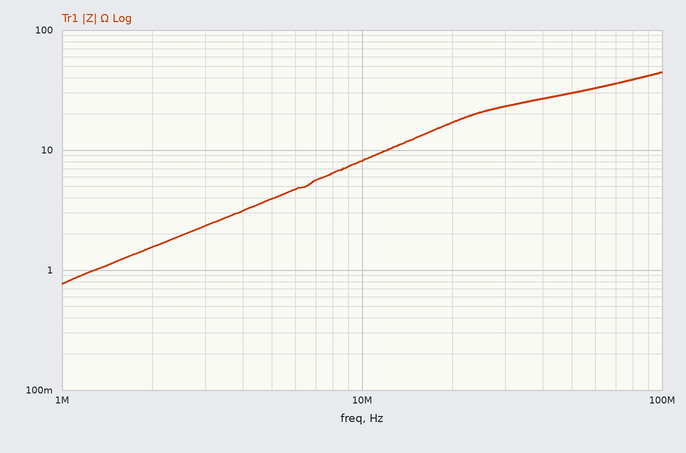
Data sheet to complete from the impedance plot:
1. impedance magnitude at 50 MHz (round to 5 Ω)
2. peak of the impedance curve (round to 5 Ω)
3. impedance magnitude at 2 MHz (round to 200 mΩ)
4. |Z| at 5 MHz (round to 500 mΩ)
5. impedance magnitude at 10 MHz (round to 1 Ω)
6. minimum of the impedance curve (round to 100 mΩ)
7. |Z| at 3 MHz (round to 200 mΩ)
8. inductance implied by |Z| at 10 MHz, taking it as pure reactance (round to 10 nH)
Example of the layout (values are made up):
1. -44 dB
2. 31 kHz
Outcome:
1. 30 Ω
2. 45 Ω
3. 1.6 Ω
4. 4.0 Ω
5. 8 Ω
6. 800 mΩ
7. 2.4 Ω
8. 130 nH
